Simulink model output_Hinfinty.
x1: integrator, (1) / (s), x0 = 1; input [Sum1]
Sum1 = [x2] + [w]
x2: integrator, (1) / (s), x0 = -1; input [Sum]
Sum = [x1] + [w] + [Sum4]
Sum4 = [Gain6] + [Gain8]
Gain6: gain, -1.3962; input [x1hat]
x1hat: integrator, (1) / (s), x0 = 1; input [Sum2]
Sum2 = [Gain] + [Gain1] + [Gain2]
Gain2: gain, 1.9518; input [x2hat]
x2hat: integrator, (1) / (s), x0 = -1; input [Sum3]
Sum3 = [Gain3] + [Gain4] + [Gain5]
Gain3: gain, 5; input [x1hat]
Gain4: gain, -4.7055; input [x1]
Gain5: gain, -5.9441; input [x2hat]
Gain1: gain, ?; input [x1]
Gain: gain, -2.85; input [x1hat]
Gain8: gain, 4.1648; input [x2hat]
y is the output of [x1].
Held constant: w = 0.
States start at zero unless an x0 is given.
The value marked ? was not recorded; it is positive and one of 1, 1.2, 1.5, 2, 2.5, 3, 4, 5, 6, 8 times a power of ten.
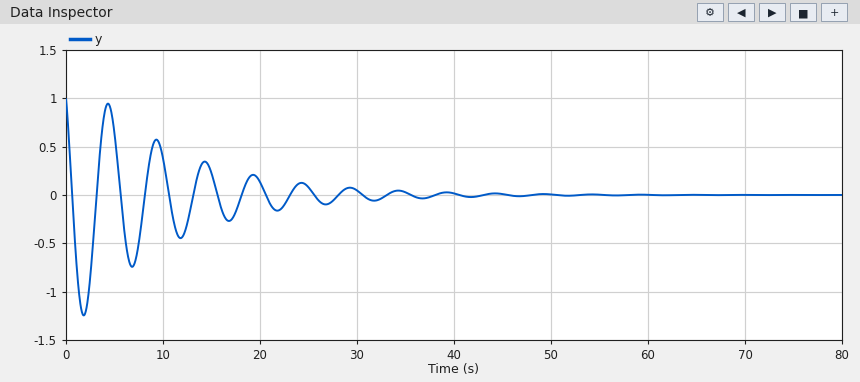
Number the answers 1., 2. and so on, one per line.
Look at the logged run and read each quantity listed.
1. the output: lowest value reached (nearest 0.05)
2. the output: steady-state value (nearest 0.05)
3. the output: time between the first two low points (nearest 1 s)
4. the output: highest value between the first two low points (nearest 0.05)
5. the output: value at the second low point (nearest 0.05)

1. -1.25
2. 0.00
3. 5 s
4. 0.95
5. -0.75
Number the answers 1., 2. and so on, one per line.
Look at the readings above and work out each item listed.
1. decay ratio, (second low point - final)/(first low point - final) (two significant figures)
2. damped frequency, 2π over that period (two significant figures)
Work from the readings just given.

1. 0.60
2. 1.3 rad/s
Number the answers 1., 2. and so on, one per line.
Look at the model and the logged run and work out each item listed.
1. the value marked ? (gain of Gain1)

1. 2.5
